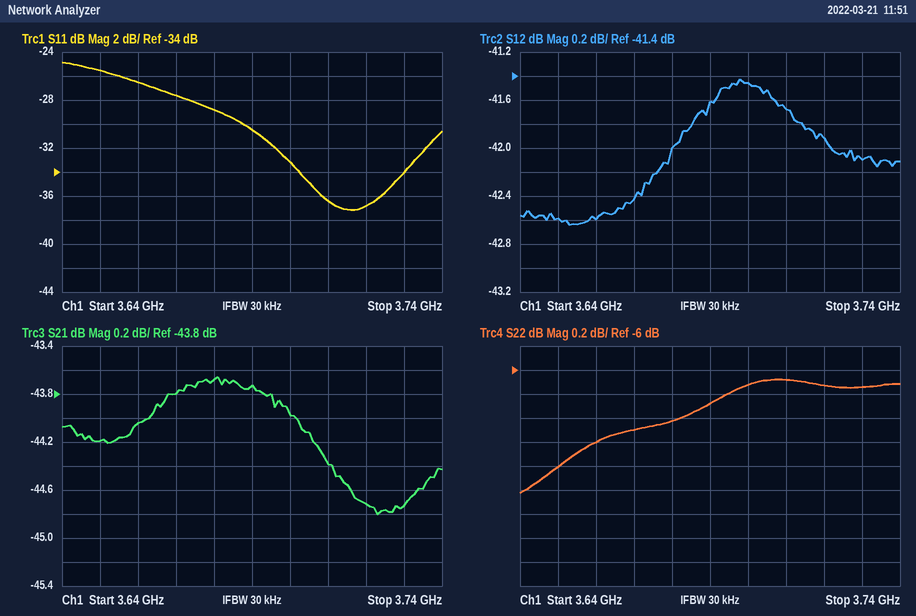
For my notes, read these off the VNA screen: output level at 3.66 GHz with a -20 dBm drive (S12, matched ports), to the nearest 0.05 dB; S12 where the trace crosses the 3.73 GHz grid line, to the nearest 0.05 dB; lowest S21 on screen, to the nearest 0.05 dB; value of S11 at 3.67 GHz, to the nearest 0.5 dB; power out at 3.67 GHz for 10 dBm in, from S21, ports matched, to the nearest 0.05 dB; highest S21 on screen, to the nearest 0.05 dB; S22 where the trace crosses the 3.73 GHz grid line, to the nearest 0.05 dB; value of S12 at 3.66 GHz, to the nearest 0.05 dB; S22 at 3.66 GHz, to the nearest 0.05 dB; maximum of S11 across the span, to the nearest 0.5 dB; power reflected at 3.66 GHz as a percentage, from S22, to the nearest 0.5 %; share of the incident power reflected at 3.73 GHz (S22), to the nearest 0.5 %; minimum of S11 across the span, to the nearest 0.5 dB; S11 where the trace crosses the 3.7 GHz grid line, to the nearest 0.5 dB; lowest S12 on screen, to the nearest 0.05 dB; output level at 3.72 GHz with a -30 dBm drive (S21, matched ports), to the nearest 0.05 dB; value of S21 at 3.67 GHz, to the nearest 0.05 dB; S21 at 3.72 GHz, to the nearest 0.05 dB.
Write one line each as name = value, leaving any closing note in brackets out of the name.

output level at 3.66 GHz with a -20 dBm drive (S12, matched ports), to the nearest 0.05 dB = -62.60 dBm
S12 where the trace crosses the 3.73 GHz grid line, to the nearest 0.05 dB = -42.10 dB
lowest S21 on screen, to the nearest 0.05 dB = -44.80 dB
value of S11 at 3.67 GHz, to the nearest 0.5 dB = -27.5 dB
power out at 3.67 GHz for 10 dBm in, from S21, ports matched, to the nearest 0.05 dB = -33.80 dBm
highest S21 on screen, to the nearest 0.05 dB = -43.65 dB
S22 where the trace crosses the 3.73 GHz grid line, to the nearest 0.05 dB = -6.15 dB
value of S12 at 3.66 GHz, to the nearest 0.05 dB = -42.60 dB
S22 at 3.66 GHz, to the nearest 0.05 dB = -6.60 dB
maximum of S11 across the span, to the nearest 0.5 dB = -25.0 dB
power reflected at 3.66 GHz as a percentage, from S22, to the nearest 0.5 % = 22.0 %
share of the incident power reflected at 3.73 GHz (S22), to the nearest 0.5 % = 24.5 %
minimum of S11 across the span, to the nearest 0.5 dB = -37.0 dB
S11 where the trace crosses the 3.7 GHz grid line, to the nearest 0.5 dB = -33.0 dB
lowest S12 on screen, to the nearest 0.05 dB = -42.65 dB
output level at 3.72 GHz with a -30 dBm drive (S21, matched ports), to the nearest 0.05 dB = -74.70 dBm
value of S21 at 3.67 GHz, to the nearest 0.05 dB = -43.80 dB
S21 at 3.72 GHz, to the nearest 0.05 dB = -44.70 dB
